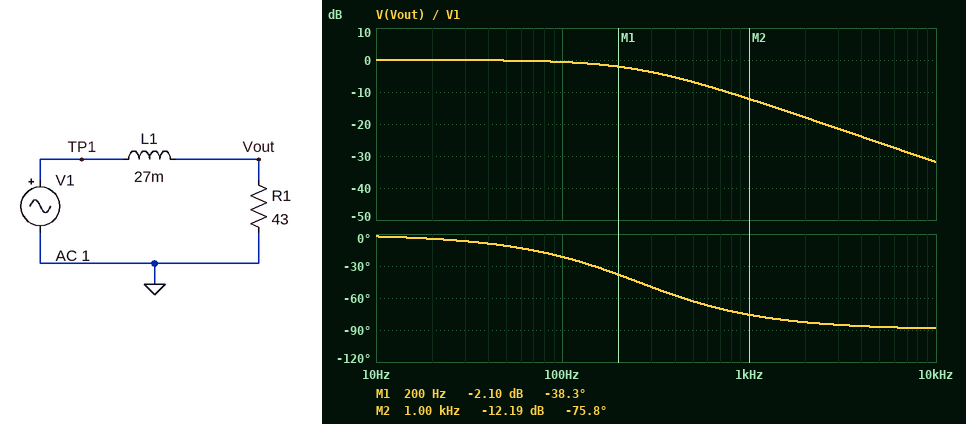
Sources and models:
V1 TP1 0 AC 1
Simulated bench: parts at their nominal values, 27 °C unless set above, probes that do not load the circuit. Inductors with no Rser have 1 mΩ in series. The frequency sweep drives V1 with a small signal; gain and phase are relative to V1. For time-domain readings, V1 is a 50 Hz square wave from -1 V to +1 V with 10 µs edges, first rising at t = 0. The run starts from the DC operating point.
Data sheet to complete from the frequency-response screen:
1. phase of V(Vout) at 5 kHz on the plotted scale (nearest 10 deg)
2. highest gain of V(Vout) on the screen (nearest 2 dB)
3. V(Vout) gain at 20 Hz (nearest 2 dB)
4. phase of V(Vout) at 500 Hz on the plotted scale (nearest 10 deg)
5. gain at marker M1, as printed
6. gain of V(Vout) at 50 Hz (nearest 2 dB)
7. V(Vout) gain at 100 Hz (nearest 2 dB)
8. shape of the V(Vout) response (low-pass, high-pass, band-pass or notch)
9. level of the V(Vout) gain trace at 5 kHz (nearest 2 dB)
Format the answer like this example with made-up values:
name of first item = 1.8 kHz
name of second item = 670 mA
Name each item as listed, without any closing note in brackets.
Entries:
phase of V(Vout) at 5 kHz on the plotted scale = -90 deg
highest gain of V(Vout) on the screen = 0 dB
V(Vout) gain at 20 Hz = 0 dB
phase of V(Vout) at 500 Hz on the plotted scale = -60 deg
gain at marker M1, as printed = -2.10 dB
gain of V(Vout) at 50 Hz = 0 dB
V(Vout) gain at 100 Hz = 0 dB
shape of the V(Vout) response = low-pass
level of the V(Vout) gain trace at 5 kHz = -26 dB
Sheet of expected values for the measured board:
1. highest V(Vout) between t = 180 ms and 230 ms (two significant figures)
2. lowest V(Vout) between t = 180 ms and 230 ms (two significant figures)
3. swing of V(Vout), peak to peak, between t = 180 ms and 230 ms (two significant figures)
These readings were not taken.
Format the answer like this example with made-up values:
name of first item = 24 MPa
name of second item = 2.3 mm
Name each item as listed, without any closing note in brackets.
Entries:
highest V(Vout) between t = 180 ms and 230 ms = 1.0 V
lowest V(Vout) between t = 180 ms and 230 ms = -1.0 V
swing of V(Vout), peak to peak, between t = 180 ms and 230 ms = 2.0 V
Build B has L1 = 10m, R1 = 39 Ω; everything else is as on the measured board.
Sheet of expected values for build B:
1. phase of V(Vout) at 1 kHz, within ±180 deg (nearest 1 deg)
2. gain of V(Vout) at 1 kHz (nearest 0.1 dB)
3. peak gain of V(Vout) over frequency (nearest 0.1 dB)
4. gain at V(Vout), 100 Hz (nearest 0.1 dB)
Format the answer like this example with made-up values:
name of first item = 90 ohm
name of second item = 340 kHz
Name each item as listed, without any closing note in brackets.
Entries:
phase of V(Vout) at 1 kHz, within ±180 deg = -58 deg
gain of V(Vout) at 1 kHz = -5.6 dB
peak gain of V(Vout) over frequency = 0 dB
gain at V(Vout), 100 Hz = -0.1 dB
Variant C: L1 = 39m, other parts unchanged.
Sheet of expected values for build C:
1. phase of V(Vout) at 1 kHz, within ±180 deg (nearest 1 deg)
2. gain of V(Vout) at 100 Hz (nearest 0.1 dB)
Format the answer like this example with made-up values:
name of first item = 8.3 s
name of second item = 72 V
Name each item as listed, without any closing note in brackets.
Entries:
phase of V(Vout) at 1 kHz, within ±180 deg = -80 deg
gain of V(Vout) at 100 Hz = -1.2 dB
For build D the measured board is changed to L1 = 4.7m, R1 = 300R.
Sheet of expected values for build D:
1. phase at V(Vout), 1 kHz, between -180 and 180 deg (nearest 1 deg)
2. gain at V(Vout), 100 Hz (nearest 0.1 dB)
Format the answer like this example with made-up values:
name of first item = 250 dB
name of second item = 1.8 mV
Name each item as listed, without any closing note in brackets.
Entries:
phase at V(Vout), 1 kHz, between -180 and 180 deg = -6 deg
gain at V(Vout), 100 Hz = 0 dB
